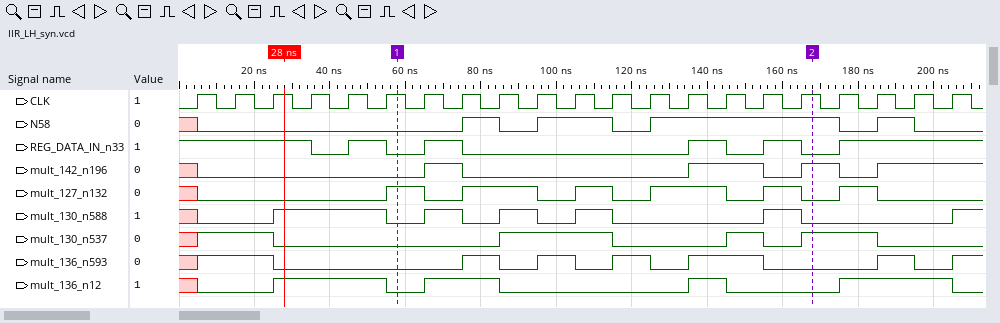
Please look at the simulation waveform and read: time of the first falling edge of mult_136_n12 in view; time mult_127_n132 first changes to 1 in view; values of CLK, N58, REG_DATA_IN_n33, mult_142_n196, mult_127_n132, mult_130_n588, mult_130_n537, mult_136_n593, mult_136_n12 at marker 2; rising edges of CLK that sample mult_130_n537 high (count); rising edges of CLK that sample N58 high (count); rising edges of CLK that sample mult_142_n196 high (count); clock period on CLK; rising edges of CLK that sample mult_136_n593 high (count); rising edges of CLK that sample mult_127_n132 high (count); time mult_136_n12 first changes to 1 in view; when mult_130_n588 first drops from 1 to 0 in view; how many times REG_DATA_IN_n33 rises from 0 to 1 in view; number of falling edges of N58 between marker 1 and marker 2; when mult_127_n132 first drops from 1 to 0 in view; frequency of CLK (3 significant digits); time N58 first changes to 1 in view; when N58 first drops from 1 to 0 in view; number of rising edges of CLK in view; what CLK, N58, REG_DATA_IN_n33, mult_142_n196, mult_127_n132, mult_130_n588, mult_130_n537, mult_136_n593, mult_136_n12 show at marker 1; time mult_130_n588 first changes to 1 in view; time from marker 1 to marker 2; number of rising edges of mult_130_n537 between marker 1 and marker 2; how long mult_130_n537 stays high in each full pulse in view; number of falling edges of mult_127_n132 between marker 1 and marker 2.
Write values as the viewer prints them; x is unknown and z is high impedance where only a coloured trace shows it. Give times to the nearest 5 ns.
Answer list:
55 ns
55 ns
CLK=1, N58=1, REG_DATA_IN_n33=0, mult_142_n196=1, mult_127_n132=0, mult_130_n588=0, mult_130_n537=1, mult_136_n593=0, mult_136_n12=0
8
9
6
10 ns
8
8
25 ns
55 ns
5
2
65 ns
100 MHz
75 ns
85 ns
21
CLK=1, N58=0, REG_DATA_IN_n33=0, mult_142_n196=0, mult_127_n132=1, mult_130_n588=0, mult_130_n537=0, mult_136_n593=0, mult_136_n12=0
25 ns
110 ns
3
30 ns, 10 ns, 20 ns
5
